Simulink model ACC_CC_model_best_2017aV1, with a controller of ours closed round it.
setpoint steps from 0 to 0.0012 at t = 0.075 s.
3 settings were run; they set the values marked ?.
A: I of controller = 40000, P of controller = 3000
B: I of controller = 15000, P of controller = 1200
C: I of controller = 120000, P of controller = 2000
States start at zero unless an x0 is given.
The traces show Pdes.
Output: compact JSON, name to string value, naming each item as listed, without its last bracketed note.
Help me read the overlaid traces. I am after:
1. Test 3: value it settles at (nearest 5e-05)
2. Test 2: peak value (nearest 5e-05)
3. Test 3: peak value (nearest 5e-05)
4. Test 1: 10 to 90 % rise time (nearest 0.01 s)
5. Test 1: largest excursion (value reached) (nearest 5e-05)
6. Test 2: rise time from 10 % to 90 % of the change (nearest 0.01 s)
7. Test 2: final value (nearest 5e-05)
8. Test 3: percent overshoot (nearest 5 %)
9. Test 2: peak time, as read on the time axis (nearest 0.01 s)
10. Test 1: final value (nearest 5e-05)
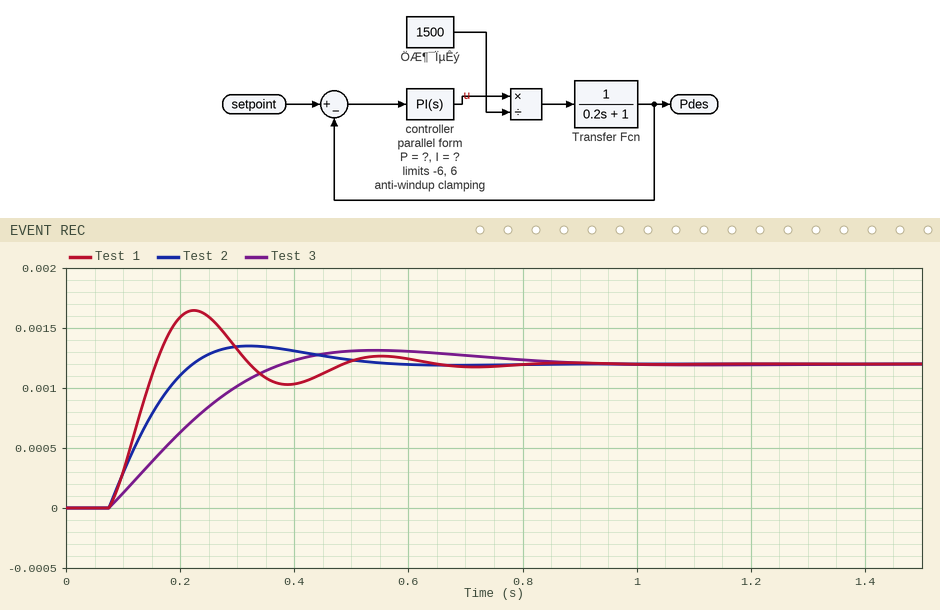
{"Test 3: value it settles at": "0.00120", "Test 2: peak value": "0.00135", "Test 3: peak value": "0.00130", "Test 1: 10 to 90 % rise time": "0.06 s", "Test 1: largest excursion (value reached)": "0.00165", "Test 2: rise time from 10 % to 90 % of the change": "0.11 s", "Test 2: final value": "0.00120", "Test 3: percent overshoot": "10 %", "Test 2: peak time, as read on the time axis": "0.32 s", "Test 1: final value": "0.00120"}
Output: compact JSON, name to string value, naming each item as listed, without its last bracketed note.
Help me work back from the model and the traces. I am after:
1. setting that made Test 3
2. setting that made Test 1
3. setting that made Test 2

{"setting that made Test 3": "B", "setting that made Test 1": "C", "setting that made Test 2": "A"}
